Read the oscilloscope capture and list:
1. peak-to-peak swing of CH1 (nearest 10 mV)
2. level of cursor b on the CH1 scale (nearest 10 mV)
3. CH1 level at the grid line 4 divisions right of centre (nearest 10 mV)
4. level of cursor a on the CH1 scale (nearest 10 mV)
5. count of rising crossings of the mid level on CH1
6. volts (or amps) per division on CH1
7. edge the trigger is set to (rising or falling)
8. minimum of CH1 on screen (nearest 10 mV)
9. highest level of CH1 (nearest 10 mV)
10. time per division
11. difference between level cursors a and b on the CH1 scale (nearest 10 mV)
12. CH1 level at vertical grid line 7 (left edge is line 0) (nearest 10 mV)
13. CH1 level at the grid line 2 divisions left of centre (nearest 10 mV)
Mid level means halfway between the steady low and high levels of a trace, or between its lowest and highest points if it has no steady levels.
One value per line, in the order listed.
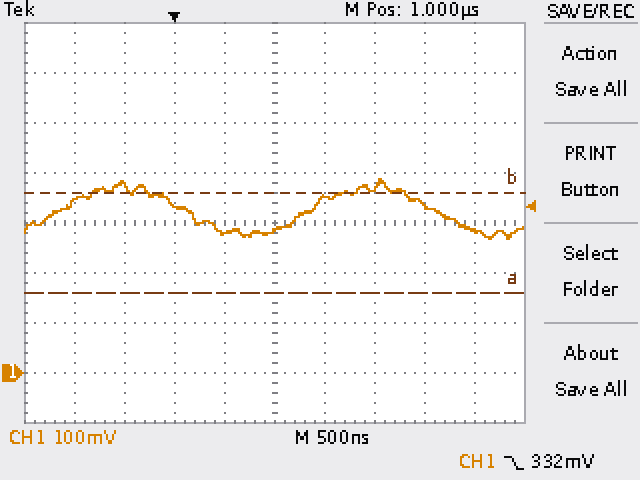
120 mV
360 mV
280 mV
160 mV
2
100 mV
falling
270 mV
390 mV
500 ns
200 mV
370 mV
330 mV
